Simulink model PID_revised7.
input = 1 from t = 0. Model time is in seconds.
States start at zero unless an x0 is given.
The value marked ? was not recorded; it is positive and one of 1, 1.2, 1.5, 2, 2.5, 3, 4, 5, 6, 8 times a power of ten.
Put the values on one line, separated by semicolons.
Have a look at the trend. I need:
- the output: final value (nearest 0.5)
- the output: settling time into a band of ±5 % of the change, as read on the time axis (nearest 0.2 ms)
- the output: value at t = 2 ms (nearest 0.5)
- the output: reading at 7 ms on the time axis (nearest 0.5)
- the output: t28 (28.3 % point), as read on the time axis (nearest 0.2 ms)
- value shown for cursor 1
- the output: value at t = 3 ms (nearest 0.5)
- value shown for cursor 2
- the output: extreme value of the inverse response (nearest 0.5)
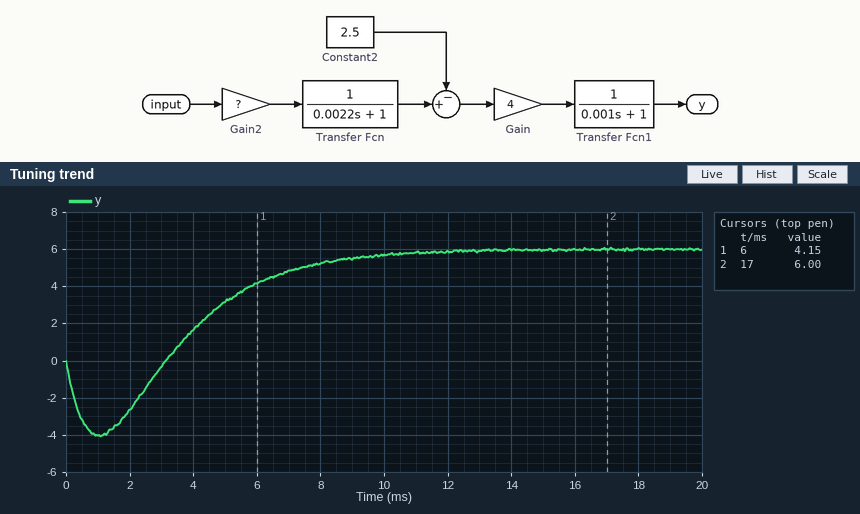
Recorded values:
6.0; 10.0 ms; -2.5; 5.0; 4.0 ms; 4.15; -0.5; 6.00; -4.0
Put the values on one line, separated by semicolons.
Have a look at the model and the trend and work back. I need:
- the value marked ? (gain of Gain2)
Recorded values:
4
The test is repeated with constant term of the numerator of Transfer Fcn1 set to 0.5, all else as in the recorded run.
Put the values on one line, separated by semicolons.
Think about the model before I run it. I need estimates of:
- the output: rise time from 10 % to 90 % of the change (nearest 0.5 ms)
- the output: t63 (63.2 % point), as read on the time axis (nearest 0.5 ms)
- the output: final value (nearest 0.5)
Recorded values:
5.0 ms; 5.5 ms; 3.0
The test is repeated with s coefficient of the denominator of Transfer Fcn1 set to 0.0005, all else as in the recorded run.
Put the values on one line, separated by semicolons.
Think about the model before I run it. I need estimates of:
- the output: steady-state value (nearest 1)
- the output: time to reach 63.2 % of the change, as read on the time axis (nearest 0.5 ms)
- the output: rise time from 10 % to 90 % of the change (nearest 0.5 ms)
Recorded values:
6; 5.0 ms; 5.0 ms
